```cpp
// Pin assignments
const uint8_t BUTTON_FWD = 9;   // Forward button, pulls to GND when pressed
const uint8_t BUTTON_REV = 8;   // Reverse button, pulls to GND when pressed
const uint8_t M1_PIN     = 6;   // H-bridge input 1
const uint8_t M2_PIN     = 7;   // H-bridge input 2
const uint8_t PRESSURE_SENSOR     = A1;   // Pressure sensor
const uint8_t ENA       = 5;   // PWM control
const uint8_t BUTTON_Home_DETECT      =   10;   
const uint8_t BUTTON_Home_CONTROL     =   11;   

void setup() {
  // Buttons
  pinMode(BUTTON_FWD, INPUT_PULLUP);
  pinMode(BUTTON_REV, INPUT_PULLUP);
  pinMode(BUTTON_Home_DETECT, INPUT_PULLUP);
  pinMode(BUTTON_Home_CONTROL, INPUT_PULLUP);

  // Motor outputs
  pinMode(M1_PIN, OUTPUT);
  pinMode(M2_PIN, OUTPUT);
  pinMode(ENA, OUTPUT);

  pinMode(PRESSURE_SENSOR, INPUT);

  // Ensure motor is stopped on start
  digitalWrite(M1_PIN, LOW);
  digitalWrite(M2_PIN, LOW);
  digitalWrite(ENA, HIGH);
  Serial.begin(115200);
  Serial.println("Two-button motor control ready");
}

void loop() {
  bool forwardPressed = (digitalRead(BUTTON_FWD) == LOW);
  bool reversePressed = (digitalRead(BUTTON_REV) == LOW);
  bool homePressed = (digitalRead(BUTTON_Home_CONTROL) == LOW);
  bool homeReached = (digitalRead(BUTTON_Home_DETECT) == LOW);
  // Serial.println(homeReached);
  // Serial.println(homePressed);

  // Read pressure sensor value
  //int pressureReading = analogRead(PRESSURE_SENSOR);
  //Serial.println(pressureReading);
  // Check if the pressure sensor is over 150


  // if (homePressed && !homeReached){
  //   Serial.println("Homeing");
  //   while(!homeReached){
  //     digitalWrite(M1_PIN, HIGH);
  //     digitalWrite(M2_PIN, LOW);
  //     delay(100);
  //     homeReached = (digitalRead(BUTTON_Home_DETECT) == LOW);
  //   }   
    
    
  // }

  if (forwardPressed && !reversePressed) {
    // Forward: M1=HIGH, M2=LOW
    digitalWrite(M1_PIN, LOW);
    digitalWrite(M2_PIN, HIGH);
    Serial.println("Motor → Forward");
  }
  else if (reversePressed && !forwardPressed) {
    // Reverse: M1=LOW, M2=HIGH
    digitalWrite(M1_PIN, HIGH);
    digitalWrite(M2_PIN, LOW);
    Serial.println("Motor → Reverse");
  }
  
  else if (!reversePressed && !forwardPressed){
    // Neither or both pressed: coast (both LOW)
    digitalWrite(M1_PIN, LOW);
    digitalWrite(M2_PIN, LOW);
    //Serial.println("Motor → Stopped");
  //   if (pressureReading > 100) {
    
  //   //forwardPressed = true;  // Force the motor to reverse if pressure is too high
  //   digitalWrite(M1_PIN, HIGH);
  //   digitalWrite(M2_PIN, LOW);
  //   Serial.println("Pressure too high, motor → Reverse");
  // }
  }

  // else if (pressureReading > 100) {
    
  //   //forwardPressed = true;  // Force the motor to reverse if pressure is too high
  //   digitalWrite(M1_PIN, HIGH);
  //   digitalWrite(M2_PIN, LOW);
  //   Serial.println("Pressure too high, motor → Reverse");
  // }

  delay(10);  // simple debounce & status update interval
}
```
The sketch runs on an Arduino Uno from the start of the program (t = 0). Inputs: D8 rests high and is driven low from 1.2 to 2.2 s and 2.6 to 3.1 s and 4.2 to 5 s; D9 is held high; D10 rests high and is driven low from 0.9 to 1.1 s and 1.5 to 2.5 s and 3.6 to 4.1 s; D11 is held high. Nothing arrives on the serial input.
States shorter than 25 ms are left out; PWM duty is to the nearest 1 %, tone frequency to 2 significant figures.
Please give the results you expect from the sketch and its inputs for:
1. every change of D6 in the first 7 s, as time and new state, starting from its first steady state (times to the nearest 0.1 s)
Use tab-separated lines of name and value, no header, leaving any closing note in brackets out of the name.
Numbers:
every change of D6 in the first 7 s, as time and new state, starting from its first steady state	0 s low; 1.2 s high; 2.2 s low; 2.6 s high; 3.1 s low; 4.2 s high; 5 s low
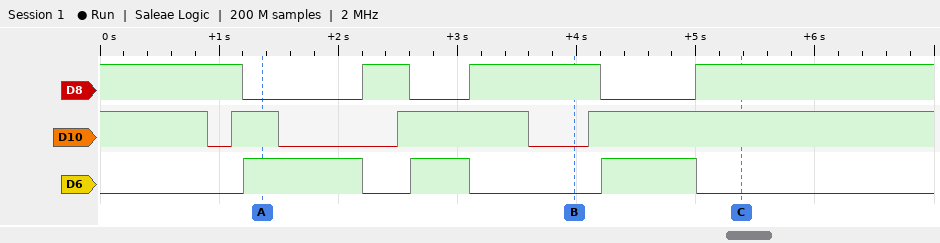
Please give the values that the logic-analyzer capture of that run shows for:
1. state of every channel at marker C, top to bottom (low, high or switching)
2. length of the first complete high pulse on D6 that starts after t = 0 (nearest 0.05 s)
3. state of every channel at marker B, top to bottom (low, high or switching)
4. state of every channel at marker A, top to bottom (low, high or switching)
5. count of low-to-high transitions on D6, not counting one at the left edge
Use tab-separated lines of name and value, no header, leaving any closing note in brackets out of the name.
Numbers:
state of every channel at marker C, top to bottom	D8 high, D10 high, D6 low
length of the first complete high pulse on D6 that starts after t = 0	1.00 s
state of every channel at marker B, top to bottom	D8 high, D10 low, D6 low
state of every channel at marker A, top to bottom	D8 low, D10 high, D6 high
count of low-to-high transitions on D6, not counting one at the left edge	3
